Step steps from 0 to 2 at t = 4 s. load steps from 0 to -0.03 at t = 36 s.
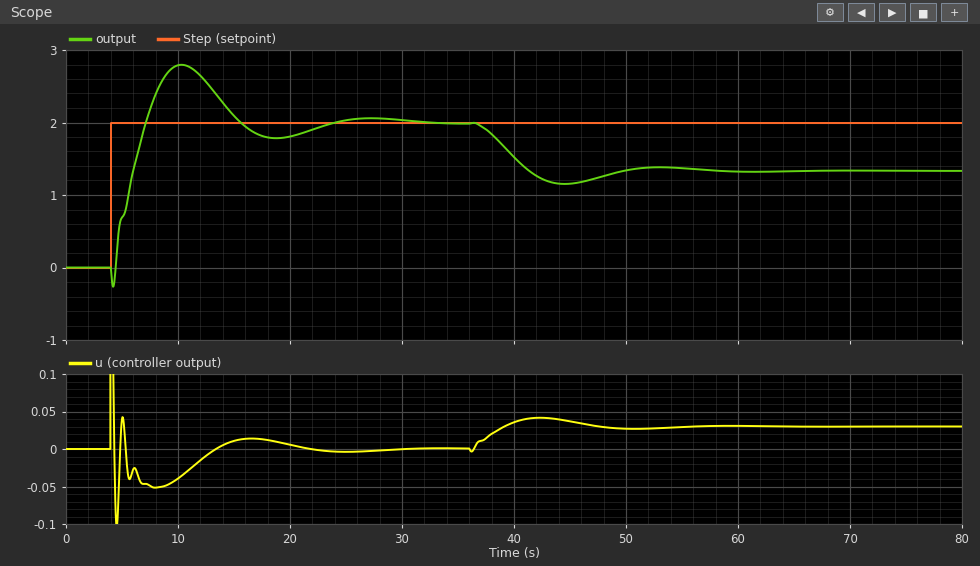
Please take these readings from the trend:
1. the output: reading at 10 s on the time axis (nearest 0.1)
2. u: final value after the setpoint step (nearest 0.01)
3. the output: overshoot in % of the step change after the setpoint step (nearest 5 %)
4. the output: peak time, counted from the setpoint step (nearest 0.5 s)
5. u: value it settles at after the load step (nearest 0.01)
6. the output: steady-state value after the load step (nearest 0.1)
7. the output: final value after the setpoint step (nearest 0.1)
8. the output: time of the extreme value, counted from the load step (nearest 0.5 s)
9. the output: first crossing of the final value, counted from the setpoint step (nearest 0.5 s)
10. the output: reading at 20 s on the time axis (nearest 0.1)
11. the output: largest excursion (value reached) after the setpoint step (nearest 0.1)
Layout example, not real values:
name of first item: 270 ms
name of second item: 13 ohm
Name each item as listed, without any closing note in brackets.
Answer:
the output: reading at 10 s on the time axis: 2.8
u: final value after the setpoint step: 0.00
the output: overshoot in % of the step change after the setpoint step: 40 %
the output: peak time, counted from the setpoint step: 6.5 s
u: value it settles at after the load step: 0.03
the output: steady-state value after the load step: 1.3
the output: final value after the setpoint step: 2.0
the output: time of the extreme value, counted from the load step: 8.5 s
the output: first crossing of the final value, counted from the setpoint step: 3.0 s
the output: reading at 20 s on the time axis: 1.8
the output: largest excursion (value reached) after the setpoint step: 2.8
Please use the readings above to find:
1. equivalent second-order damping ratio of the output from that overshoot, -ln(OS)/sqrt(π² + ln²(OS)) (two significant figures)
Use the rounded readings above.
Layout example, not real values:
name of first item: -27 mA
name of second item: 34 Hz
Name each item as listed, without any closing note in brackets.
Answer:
equivalent second-order damping ratio of the output from that overshoot, -ln(OS)/sqrt(π² + ln²(OS)): 0.28
